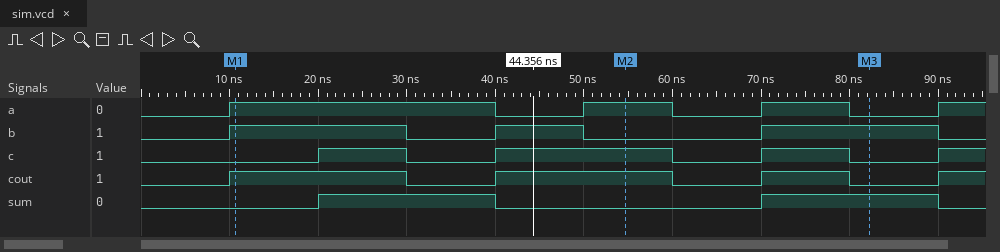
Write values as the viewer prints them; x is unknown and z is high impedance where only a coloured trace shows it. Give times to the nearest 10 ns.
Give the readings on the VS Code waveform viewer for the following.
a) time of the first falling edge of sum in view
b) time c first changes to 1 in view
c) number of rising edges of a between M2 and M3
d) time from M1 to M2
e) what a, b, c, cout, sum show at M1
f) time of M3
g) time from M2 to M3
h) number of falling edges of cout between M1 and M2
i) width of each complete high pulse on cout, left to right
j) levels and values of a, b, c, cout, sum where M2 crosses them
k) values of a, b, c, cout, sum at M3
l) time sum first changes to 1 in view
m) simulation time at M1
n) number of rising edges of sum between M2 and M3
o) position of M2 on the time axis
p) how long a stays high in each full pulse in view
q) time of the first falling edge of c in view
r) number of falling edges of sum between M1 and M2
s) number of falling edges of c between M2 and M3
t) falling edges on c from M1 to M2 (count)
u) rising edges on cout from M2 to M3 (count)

40 ns
20 ns
1
40 ns
a=1, b=1, c=0, cout=1, sum=0
80 ns
30 ns
1
20 ns, 20 ns, 10 ns
a=1, b=0, c=1, cout=1, sum=0
a=0, b=1, c=0, cout=0, sum=1
20 ns
10 ns
1
50 ns
30 ns, 10 ns, 10 ns
30 ns
1
2
1
1
